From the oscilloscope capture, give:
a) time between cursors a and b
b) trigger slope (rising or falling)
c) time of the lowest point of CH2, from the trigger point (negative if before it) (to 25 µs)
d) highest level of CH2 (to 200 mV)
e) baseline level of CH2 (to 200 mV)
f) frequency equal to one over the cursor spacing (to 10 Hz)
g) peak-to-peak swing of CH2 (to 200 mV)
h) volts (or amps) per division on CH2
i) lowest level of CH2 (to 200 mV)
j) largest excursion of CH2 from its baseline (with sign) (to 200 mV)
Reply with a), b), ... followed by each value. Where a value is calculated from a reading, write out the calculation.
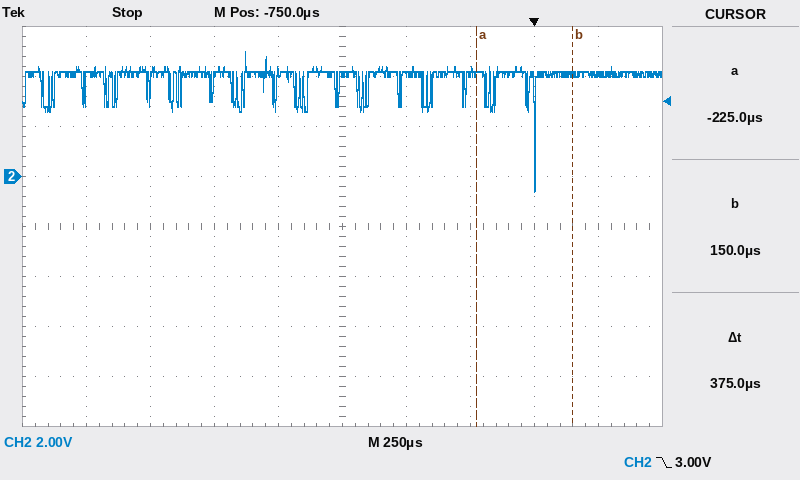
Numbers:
a) 375 µs
b) falling
c) 0 µs
d) 5.0 V
e) 4.2 V
f) 1 / 375 µs ≈ 2.67 kHz
g) 5.0 V − (-600 mV) = 5.6 V
h) 2 V
i) -600 mV
j) -600 mV − (4.2 V) = -4.8 V
